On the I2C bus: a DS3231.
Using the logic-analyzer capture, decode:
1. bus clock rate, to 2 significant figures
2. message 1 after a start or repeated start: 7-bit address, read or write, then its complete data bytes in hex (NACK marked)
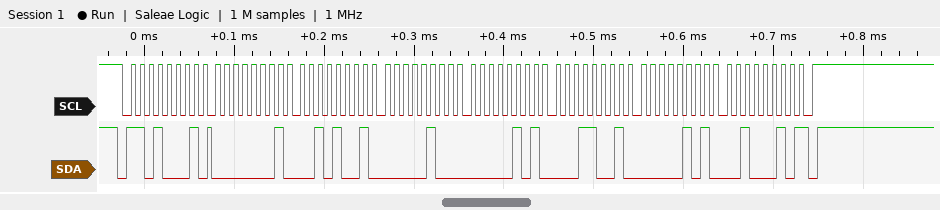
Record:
100 kHz
0x68 read: 01 29 04 05 19 05 22 NACK
